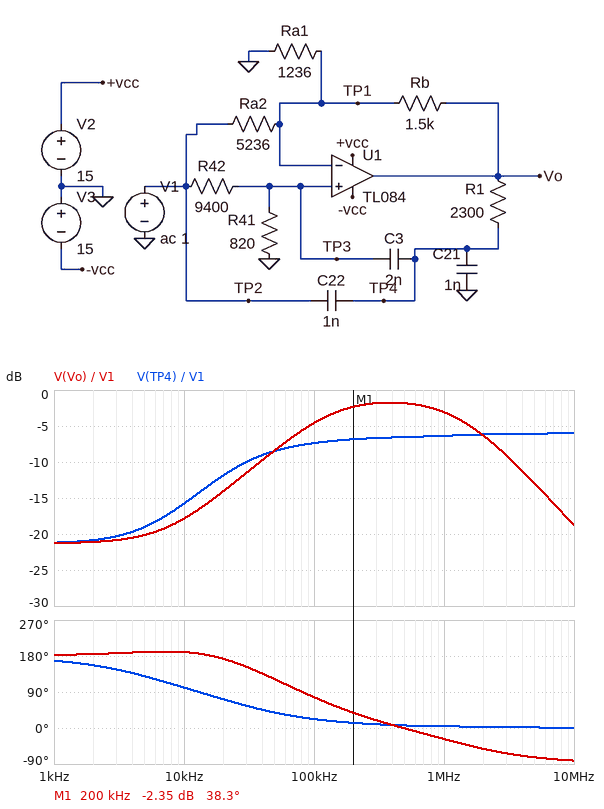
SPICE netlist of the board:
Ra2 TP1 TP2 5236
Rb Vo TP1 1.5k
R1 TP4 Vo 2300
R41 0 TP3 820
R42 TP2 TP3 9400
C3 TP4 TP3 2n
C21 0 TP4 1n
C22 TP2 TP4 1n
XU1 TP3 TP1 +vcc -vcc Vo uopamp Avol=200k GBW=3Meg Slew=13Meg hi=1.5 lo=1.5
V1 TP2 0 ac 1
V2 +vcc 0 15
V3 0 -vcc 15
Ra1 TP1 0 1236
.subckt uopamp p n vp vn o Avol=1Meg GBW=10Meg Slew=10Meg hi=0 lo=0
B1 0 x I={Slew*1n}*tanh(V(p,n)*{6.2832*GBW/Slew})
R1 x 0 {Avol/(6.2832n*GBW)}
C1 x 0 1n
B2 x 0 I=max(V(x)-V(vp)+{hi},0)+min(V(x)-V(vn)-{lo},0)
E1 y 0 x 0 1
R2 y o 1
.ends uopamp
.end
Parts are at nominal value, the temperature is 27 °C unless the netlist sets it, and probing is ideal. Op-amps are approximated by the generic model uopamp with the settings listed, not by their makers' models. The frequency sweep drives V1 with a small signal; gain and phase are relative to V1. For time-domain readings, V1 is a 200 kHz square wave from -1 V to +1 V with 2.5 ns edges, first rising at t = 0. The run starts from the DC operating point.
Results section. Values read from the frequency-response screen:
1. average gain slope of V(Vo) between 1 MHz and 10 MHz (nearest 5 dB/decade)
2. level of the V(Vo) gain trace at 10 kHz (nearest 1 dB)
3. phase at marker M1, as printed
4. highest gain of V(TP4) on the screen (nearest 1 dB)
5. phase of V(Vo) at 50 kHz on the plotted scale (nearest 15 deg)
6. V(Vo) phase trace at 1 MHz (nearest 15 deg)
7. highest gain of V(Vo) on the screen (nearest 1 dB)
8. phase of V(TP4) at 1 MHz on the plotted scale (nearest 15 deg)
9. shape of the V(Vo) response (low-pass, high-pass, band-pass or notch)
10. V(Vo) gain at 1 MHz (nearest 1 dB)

-15 dB/decade
-18 dB
38.3 deg
-6 dB
120 deg
-30 deg
-2 dB
0 deg
band-pass
-3 dB
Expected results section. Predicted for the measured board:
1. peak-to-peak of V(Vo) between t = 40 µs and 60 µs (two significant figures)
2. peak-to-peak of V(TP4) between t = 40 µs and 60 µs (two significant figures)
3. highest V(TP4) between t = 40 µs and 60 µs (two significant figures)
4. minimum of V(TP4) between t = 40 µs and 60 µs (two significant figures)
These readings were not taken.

2.7 V
1.4 V
690 mV
-690 mV
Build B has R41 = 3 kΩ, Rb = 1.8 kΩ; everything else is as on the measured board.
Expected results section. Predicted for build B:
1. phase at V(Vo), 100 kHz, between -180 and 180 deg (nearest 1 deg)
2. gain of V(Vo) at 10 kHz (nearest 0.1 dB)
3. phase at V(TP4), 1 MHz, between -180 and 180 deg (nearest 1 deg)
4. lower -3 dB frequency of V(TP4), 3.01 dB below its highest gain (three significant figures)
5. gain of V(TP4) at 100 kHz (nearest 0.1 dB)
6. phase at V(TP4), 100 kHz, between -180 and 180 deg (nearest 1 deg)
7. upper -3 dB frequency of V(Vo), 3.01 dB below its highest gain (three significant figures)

-7 deg
-10.8 dB
1 deg
30.3 kHz
-5.9 dB
-11 deg
39.0 kHz
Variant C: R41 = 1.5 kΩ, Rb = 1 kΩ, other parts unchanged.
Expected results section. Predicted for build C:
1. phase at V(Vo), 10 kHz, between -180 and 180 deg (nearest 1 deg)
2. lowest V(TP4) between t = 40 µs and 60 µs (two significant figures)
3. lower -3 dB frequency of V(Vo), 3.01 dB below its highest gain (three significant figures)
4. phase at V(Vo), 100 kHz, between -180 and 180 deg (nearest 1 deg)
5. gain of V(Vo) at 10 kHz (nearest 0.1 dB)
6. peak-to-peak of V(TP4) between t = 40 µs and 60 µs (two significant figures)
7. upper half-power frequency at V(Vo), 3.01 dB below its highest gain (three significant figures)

-3 deg
-600 mV
65.3 kHz
40 deg
-26.4 dB
1.2 V
1.69 MHz
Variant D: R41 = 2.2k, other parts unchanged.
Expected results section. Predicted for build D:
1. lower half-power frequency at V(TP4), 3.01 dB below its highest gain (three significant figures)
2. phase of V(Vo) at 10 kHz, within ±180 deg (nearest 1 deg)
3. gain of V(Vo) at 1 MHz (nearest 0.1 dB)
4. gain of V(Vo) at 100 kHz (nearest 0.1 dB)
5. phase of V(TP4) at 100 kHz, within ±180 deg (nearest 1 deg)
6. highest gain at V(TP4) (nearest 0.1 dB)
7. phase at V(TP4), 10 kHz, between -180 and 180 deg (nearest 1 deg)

28.0 kHz
4 deg
-3.0 dB
-0.5 dB
-1 deg
-3.6 dB
26 deg
